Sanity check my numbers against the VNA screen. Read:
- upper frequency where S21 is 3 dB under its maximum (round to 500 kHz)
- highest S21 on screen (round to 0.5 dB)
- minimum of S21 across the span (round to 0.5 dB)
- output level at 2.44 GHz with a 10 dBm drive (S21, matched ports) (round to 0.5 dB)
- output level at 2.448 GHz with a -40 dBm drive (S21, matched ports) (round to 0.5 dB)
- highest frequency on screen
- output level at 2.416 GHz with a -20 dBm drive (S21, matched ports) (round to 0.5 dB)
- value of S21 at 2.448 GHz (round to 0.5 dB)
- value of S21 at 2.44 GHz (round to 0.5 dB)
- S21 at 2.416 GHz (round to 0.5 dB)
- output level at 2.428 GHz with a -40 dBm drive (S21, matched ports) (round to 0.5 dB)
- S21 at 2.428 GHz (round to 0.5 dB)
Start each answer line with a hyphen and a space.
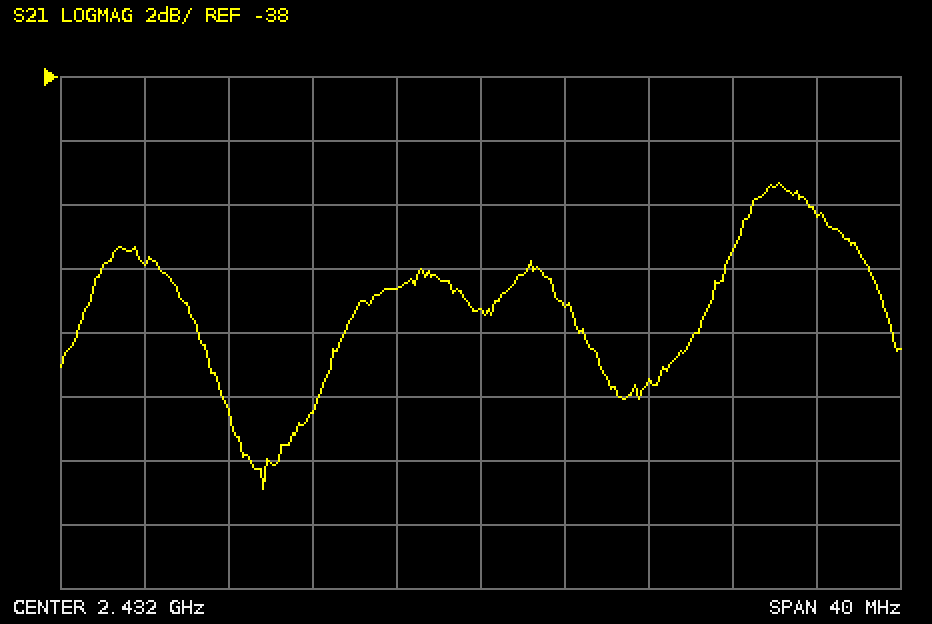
- 2.4505 GHz
- -41.5 dB
- -51.0 dB
- -37.5 dBm
- -82.5 dBm
- 2.452 GHz
- -64.0 dBm
- -42.5 dB
- -47.5 dB
- -44.0 dB
- -84.5 dBm
- -44.5 dB
